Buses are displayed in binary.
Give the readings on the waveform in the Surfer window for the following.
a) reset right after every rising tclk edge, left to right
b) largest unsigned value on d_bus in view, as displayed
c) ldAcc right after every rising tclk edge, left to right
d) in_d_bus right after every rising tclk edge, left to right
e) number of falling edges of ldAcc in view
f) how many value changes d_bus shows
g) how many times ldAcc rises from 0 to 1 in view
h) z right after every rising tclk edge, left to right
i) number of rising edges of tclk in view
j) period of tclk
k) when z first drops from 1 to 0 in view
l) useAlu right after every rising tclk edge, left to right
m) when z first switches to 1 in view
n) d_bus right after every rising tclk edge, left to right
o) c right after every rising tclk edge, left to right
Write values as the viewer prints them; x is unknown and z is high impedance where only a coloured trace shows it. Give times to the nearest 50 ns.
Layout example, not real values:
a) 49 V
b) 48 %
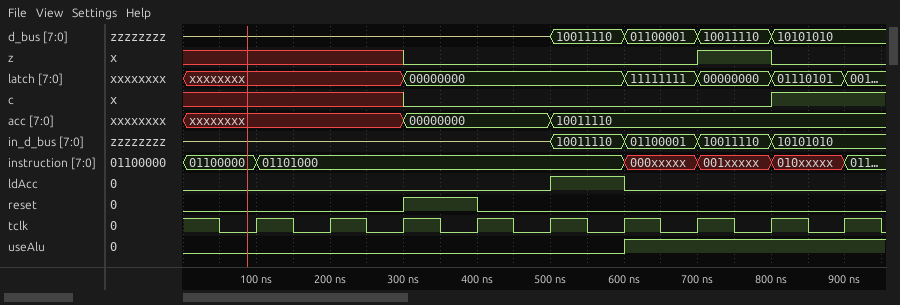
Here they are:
a) 0 0 1 0 0 0 0 0 0
b) 10101010
c) 0 0 0 0 1 0 0 0 0
d) z, z, z, z, 10011110, 01100001, 10011110, 10101010, 10101010
e) 1
f) 4
g) 1
h) x x 0 0 0 0 1 0 0
i) 9
j) 100 ns
k) 800 ns
l) 0 0 0 0 0 1 1 1 1
m) 700 ns
n) z, z, z, z, 10011110, 01100001, 10011110, 10101010, 10101010
o) x x 0 0 0 0 0 1 1
